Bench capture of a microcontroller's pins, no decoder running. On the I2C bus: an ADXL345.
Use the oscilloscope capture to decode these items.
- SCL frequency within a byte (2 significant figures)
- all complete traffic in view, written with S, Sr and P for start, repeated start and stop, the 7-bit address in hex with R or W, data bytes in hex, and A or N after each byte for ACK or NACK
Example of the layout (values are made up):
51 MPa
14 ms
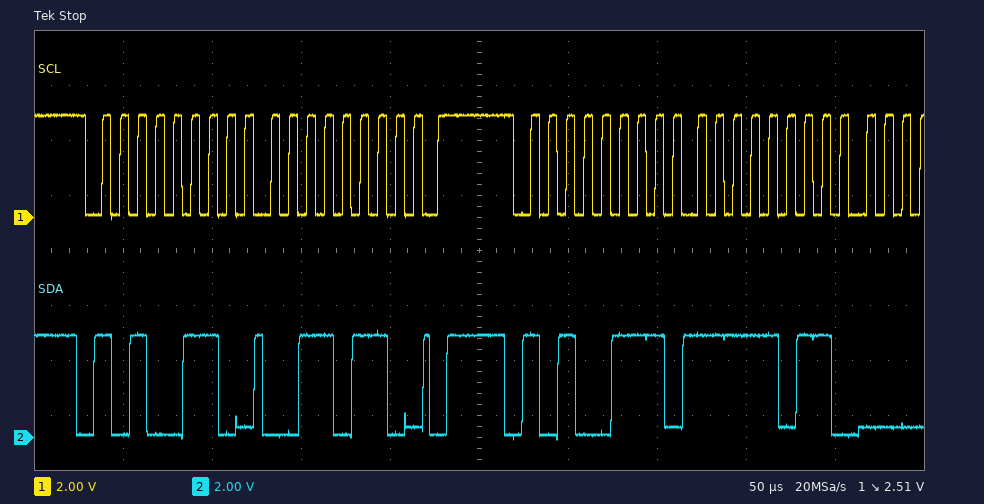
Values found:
100 kHz
S 53W A 36 A P S 53R A FB A
